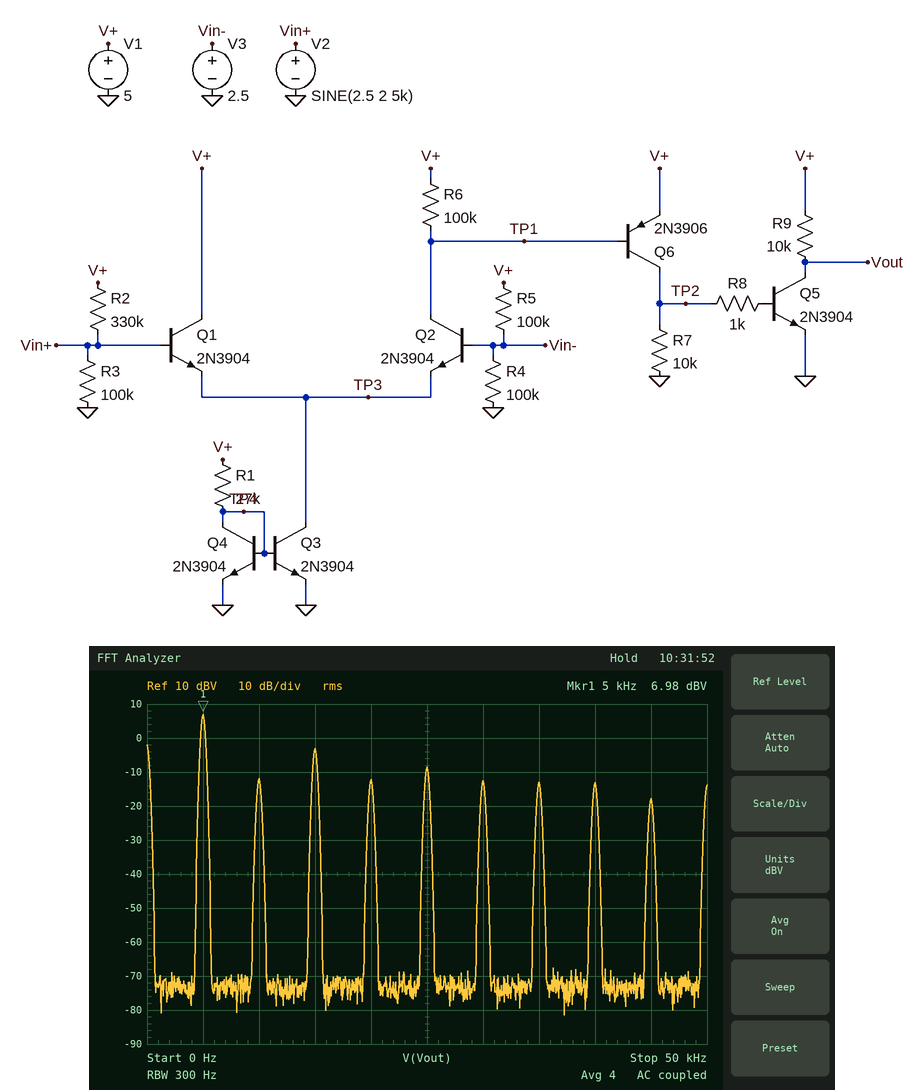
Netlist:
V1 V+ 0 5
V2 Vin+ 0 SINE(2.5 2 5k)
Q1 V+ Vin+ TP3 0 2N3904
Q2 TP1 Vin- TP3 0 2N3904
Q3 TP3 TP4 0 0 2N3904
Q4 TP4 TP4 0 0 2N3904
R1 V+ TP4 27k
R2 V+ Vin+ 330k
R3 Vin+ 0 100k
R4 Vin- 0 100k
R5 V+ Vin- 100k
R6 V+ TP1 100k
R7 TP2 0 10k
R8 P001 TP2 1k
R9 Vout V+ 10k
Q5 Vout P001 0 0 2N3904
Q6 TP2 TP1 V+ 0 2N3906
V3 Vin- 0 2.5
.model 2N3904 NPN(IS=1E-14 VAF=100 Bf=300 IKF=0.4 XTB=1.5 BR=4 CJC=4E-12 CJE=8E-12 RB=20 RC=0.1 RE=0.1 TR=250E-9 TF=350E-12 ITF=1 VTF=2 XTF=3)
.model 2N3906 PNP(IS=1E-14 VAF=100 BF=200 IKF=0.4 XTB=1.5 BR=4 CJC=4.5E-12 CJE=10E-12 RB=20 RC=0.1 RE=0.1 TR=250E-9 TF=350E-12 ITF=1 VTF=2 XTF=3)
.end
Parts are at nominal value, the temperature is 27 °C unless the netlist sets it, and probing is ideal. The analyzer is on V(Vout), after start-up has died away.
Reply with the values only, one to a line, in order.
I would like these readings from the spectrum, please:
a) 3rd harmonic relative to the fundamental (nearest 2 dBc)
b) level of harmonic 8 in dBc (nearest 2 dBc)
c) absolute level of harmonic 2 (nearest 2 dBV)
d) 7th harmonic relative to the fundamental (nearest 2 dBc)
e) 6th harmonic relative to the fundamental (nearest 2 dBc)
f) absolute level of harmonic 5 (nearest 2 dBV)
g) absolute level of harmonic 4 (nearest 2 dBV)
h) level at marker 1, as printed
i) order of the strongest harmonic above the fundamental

-10 dBc
-20 dBc
-12 dBV
-20 dBc
-20 dBc
-8 dBV
-12 dBV
6.98 dBV
3
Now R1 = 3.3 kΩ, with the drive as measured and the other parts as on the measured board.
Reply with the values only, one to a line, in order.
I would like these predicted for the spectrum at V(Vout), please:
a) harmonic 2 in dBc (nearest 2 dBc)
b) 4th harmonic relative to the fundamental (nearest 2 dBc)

-16 dBc
-16 dBc
